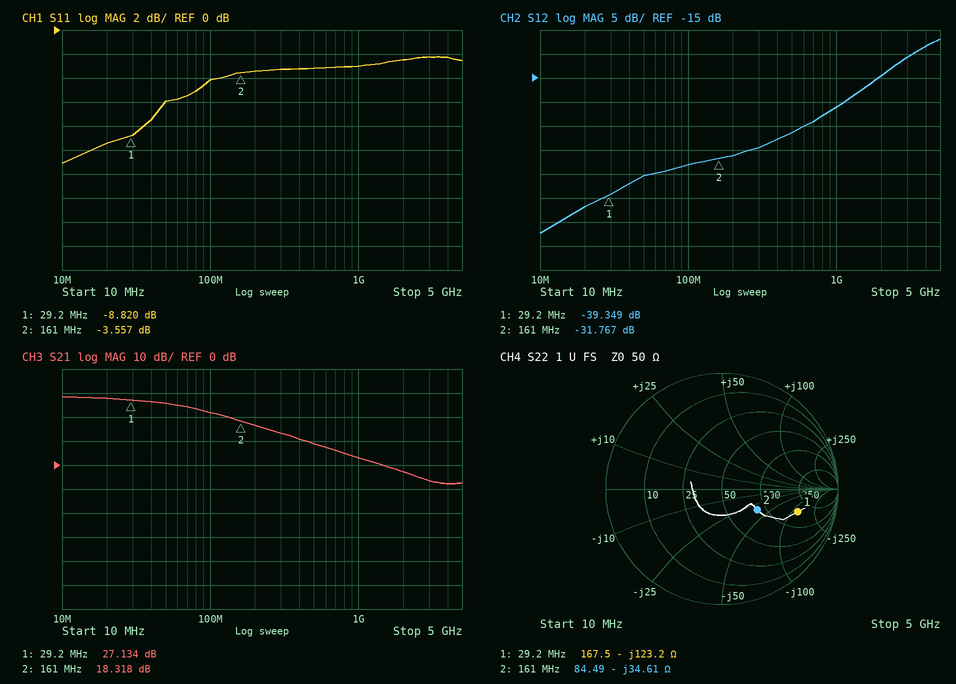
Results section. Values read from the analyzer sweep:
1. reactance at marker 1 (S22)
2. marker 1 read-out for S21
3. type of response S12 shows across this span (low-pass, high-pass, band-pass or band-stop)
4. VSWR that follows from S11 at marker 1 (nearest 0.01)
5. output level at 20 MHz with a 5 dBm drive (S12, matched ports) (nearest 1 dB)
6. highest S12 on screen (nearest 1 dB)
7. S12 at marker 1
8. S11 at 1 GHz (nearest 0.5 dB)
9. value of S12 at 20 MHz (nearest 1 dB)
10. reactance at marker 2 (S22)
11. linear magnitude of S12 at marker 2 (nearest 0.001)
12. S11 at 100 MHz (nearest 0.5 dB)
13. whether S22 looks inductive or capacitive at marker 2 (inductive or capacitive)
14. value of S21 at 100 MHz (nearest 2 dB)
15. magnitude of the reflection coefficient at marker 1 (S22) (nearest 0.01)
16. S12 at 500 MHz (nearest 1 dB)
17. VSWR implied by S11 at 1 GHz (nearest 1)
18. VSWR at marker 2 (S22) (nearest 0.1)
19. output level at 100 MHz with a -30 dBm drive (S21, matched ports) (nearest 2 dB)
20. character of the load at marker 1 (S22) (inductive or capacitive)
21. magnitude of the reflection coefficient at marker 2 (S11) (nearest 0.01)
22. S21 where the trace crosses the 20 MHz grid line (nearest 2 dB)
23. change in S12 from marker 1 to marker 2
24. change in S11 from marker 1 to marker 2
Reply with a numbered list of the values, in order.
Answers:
1. -123.2 Ω
2. 27.134 dB
3. high-pass
4. 2.14
5. -37 dBm
6. -7 dB
7. -39.349 dB
8. -3.0 dB
9. -42 dB
10. -34.61 Ω
11. 0.026
12. -4.0 dB
13. capacitive
14. 22 dB
15. 0.68
16. -26 dB
17. 6
18. 2.1
19. -8 dBm
20. capacitive
21. 0.66
22. 28 dB
23. 7.582 dB
24. 5.263 dB
